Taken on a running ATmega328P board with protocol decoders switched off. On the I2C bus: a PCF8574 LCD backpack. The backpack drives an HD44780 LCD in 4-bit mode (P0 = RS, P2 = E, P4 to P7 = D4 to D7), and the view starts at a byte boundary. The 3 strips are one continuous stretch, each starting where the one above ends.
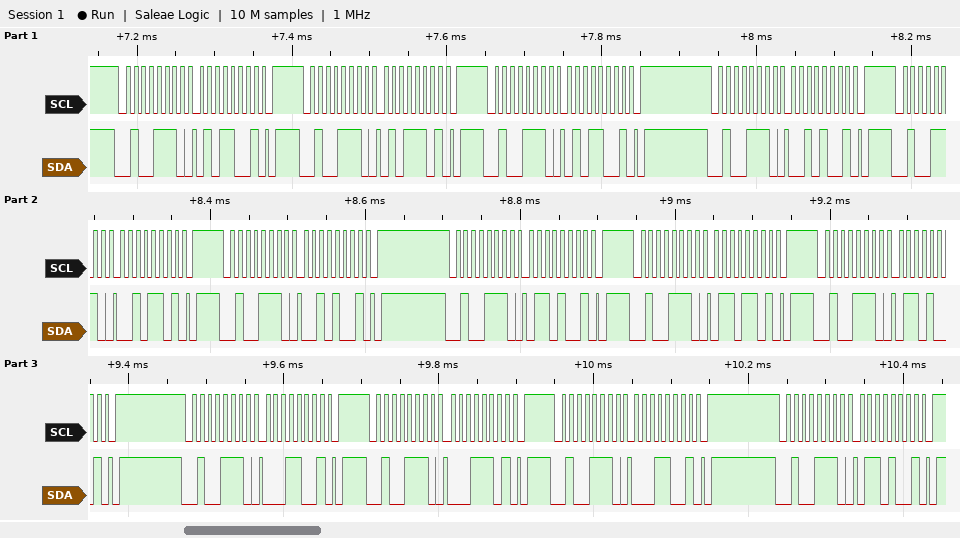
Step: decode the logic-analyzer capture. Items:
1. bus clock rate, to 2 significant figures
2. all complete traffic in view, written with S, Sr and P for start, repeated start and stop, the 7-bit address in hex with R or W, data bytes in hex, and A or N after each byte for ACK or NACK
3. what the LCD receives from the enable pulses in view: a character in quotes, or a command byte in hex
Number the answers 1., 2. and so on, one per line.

1. 100 kHz
2. S 27W A 59 A P S 27W A 5D A P S 27W A 59 A P S 27W A 29 A P S 27W A 2D A P S 27W A 29 A P S 27W A 69 A P S 27W A 6D A P S 27W A 69 A P S 27W A 19 A P S 27W A 1D A P S 27W A 19 A P S 27W A 69 A P
3. 'R' 'a'
